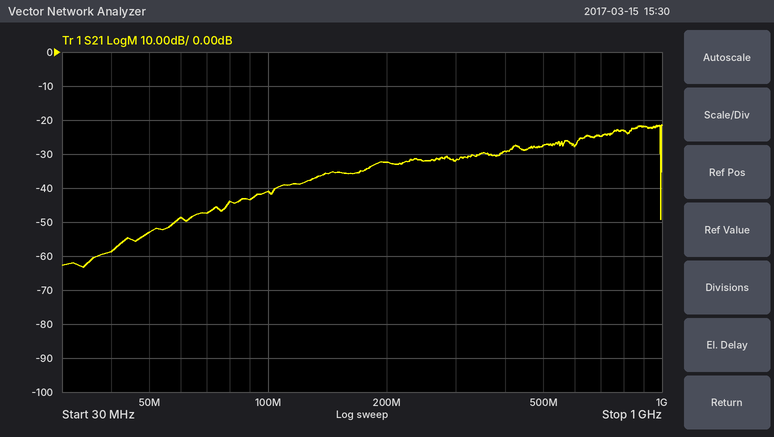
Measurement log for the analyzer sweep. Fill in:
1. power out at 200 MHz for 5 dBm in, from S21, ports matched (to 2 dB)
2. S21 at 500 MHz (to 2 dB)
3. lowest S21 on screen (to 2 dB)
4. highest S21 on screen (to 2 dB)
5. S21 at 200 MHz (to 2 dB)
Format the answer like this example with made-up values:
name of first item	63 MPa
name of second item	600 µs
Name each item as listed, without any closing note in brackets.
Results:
power out at 200 MHz for 5 dBm in, from S21, ports matched	-28 dBm
S21 at 500 MHz	-28 dB
lowest S21 on screen	-64 dB
highest S21 on screen	-22 dB
S21 at 200 MHz	-32 dB
